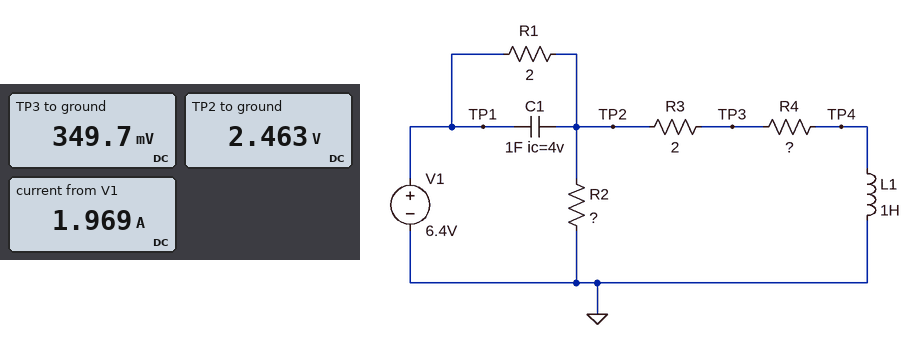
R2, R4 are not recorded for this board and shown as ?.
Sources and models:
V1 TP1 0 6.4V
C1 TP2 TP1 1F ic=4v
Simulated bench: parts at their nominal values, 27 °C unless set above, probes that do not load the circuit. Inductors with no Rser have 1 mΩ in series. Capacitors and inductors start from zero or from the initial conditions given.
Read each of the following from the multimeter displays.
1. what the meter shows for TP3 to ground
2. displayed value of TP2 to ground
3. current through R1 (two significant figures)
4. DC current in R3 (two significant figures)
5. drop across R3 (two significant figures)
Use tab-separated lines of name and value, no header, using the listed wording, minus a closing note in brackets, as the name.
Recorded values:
what the meter shows for TP3 to ground	349.7 mV
displayed value of TP2 to ground	2.463 V
current through R1	2.0 A
DC current in R3	1.1 A
drop across R3	2.1 V
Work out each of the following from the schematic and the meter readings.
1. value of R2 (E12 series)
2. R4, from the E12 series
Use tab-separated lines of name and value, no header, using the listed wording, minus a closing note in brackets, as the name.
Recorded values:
value of R2	2.7 Ω
R4, from the E12 series	0.33 Ω
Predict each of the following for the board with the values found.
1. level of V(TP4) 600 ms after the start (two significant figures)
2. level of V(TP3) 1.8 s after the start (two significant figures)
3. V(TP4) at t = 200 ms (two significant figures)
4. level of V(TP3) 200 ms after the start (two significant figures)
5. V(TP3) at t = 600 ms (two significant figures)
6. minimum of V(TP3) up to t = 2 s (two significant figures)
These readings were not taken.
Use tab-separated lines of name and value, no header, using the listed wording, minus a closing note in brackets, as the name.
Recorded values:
level of V(TP4) 600 ms after the start	460 mV
level of V(TP3) 1.8 s after the start	360 mV
V(TP4) at t = 200 ms	1.8 V
level of V(TP3) 200 ms after the start	2.0 V
V(TP3) at t = 600 ms	760 mV
minimum of V(TP3) up to t = 2 s	350 mV
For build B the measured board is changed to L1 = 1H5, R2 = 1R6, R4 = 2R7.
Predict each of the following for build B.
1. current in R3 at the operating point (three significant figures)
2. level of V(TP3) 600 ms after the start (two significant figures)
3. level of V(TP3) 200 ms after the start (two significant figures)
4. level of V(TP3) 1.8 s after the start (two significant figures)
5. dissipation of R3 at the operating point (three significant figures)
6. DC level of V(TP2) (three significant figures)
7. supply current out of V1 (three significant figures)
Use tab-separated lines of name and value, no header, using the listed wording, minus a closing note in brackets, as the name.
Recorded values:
current in R3 at the operating point	509 mA
level of V(TP3) 600 ms after the start	1.5 V
level of V(TP3) 200 ms after the start	2.1 V
level of V(TP3) 1.8 s after the start	1.4 V
dissipation of R3 at the operating point	518 mW
DC level of V(TP2)	2.39 V
supply current out of V1	2.00 A
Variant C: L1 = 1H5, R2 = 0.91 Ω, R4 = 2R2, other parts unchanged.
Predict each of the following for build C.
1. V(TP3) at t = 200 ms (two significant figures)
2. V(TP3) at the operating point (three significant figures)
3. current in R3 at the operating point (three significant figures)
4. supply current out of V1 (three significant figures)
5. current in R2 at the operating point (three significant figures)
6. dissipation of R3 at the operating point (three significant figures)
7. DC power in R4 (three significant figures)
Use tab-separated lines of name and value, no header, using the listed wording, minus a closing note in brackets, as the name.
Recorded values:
V(TP3) at t = 200 ms	1.5 V
V(TP3) at the operating point	913 mV
current in R3 at the operating point	415 mA
supply current out of V1	2.33 A
current in R2 at the operating point	1.91 A
dissipation of R3 at the operating point	344 mW
DC power in R4	378 mW
